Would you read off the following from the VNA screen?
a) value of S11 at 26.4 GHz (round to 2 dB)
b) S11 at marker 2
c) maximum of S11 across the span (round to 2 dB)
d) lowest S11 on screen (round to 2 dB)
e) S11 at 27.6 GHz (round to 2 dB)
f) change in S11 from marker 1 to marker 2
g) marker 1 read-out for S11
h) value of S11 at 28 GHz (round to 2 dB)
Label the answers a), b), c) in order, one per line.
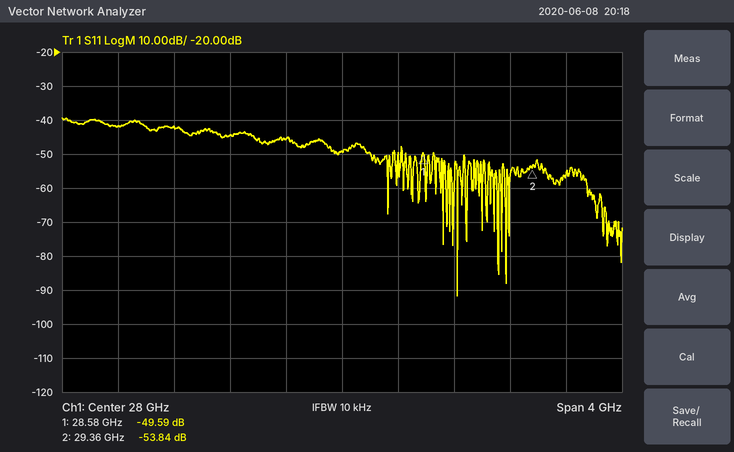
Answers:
a) -42 dB
b) -53.84 dB
c) -40 dB
d) -92 dB
e) -46 dB
f) -4.25 dB
g) -49.59 dB
h) -50 dB
